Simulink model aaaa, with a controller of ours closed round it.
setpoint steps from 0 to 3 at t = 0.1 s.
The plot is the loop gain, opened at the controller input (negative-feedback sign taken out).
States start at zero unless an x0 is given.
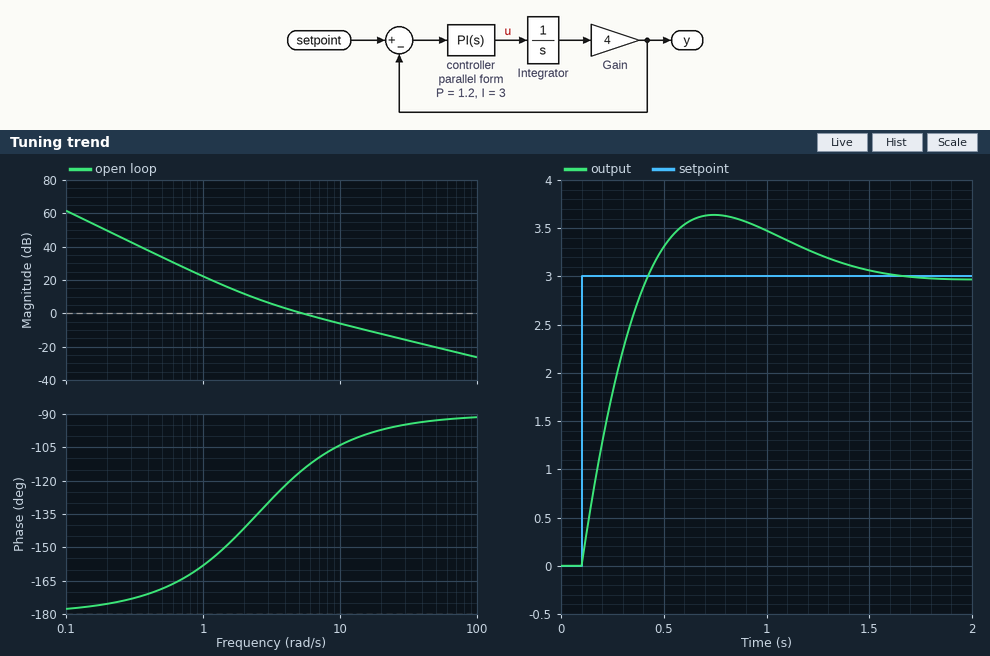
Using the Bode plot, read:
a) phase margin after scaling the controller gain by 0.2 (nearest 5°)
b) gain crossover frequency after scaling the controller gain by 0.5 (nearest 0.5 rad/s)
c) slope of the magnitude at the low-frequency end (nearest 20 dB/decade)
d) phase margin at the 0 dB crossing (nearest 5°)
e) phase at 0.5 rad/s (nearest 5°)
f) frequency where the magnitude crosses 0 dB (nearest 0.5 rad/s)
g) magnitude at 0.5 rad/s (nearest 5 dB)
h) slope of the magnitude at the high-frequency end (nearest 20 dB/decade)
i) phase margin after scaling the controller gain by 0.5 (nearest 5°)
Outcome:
35°
3.0 rad/s
-40 dB/decade
65°
-170°
5.5 rad/s
35 dB
-20 dB/decade
50°
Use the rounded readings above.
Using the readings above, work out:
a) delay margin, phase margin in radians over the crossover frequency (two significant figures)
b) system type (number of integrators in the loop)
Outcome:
0.21 s
2
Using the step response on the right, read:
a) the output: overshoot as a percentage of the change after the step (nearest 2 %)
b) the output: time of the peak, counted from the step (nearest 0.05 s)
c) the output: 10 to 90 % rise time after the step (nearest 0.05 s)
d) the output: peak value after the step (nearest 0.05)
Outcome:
22 %
0.65 s
0.25 s
3.65
